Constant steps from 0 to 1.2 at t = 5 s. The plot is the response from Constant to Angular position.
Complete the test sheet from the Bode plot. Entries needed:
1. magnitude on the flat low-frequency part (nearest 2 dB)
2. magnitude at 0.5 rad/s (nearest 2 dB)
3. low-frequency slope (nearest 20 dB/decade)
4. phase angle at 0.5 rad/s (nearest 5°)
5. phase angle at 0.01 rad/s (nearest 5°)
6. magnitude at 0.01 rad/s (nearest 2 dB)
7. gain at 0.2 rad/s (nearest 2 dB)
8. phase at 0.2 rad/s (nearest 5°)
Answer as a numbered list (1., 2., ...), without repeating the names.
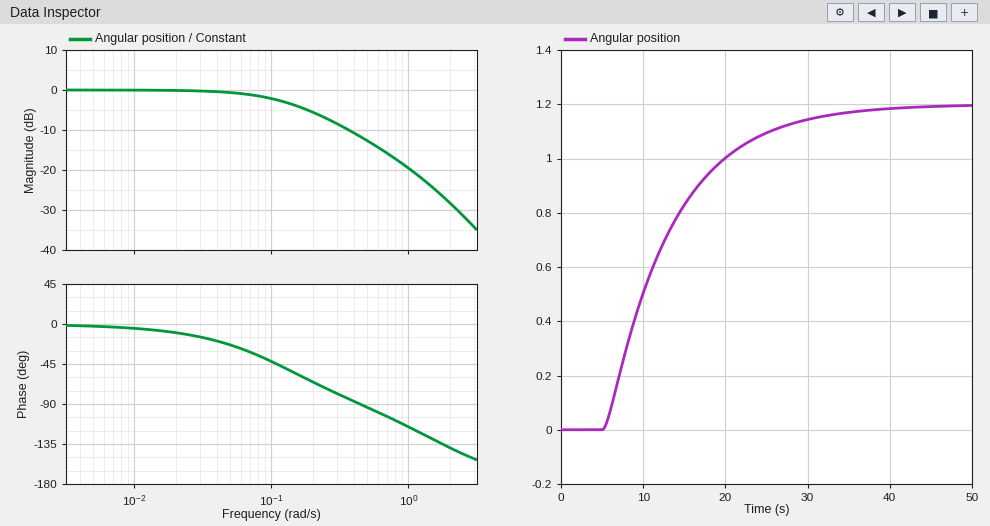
1. 0 dB
2. -12 dB
3. 0 dB/decade
4. -95°
5. -5°
6. 0 dB
7. -6 dB
8. -65°
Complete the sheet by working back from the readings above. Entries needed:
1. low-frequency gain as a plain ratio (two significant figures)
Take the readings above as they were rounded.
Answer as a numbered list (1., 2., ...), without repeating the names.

1. 1.0
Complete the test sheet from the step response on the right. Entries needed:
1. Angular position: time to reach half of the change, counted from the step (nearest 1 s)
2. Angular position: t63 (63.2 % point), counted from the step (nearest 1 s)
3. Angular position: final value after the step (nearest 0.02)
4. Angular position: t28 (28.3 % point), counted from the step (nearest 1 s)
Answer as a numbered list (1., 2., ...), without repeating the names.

1. 6 s
2. 9 s
3. 1.20
4. 3 s
